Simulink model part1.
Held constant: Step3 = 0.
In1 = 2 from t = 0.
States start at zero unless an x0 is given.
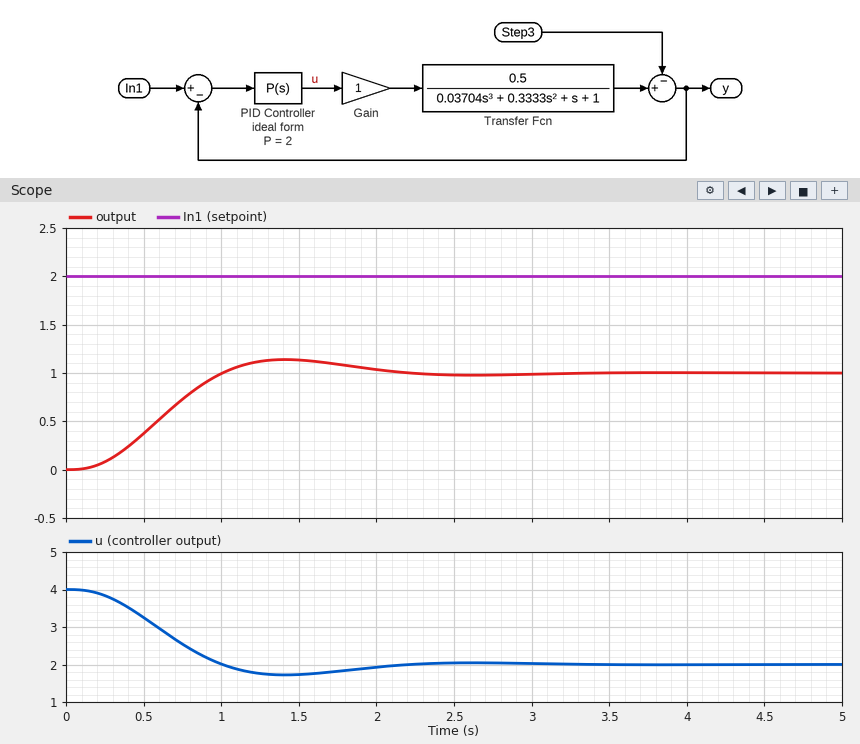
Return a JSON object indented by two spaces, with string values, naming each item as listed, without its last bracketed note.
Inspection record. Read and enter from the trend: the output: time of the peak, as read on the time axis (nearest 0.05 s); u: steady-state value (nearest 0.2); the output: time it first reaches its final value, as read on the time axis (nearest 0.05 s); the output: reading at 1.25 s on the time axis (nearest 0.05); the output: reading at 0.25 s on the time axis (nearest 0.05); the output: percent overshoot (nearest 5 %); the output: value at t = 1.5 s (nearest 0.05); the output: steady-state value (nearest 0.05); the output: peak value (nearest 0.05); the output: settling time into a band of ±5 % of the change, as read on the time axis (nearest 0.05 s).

{
  "the output: time of the peak, as read on the time axis": "1.40 s",
  "u: steady-state value": "2.0",
  "the output: time it first reaches its final value, as read on the time axis": "1.00 s",
  "the output: reading at 1.25 s on the time axis": "1.10",
  "the output: reading at 0.25 s on the time axis": "0.10",
  "the output: percent overshoot": "15 %",
  "the output: value at t = 1.5 s": "1.15",
  "the output: steady-state value": "1.00",
  "the output: peak value": "1.15",
  "the output: settling time into a band of ±5 % of the change, as read on the time axis": "1.95 s"
}
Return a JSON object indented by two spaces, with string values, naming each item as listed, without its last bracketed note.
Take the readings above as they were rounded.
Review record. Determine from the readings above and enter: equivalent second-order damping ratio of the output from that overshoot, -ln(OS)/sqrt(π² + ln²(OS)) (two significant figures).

{
  "equivalent second-order damping ratio of the output from that overshoot, -ln(OS)/sqrt(π² + ln²(OS))": "0.52"
}
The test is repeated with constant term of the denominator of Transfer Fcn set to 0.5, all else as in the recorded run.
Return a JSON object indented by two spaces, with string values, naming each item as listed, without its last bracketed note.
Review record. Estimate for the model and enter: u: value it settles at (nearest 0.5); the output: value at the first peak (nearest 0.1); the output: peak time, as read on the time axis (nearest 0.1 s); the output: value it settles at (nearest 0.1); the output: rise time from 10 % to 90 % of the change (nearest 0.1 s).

{
  "u: value it settles at": "1.5",
  "the output: value at the first peak": "1.4",
  "the output: peak time, as read on the time axis": "1.8 s",
  "the output: value it settles at": "1.3",
  "the output: rise time from 10 % to 90 % of the change": "0.8 s"
}
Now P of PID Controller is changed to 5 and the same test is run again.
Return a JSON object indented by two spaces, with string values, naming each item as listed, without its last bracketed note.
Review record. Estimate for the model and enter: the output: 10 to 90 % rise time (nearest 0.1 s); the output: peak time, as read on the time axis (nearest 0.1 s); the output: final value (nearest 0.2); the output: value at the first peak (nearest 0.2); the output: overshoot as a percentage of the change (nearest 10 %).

{
  "the output: 10 to 90 % rise time": "0.4 s",
  "the output: peak time, as read on the time axis": "1.0 s",
  "the output: final value": "1.4",
  "the output: value at the first peak": "2.0",
  "the output: overshoot as a percentage of the change": "40 %"
}
